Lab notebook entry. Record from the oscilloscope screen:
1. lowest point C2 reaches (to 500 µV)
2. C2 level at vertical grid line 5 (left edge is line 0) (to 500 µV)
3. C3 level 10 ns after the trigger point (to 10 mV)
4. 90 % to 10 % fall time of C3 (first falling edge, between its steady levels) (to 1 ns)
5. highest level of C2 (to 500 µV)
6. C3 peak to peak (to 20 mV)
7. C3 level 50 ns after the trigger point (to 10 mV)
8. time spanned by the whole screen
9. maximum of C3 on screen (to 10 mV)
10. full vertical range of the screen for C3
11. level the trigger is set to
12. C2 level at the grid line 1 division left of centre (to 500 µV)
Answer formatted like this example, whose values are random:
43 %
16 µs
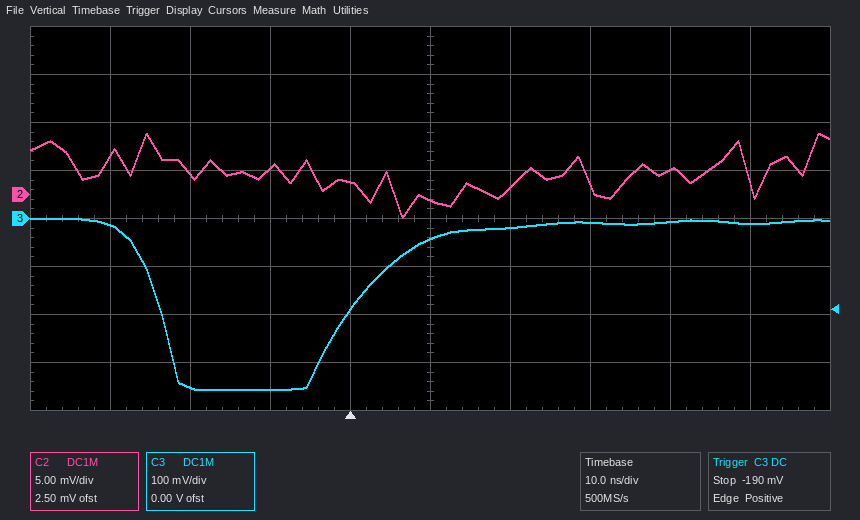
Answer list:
-2.5 mV
-500 µV
-40 mV
6 ns
6.5 mV
360 mV
-10 mV
100 ns
0 mV
800 mV
-190 mV
1.5 mV
